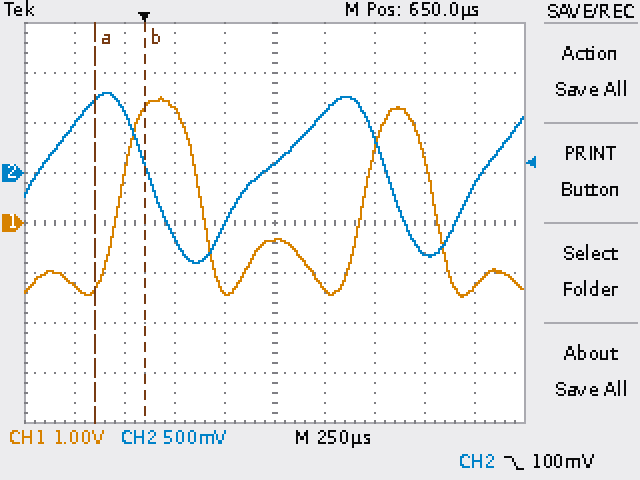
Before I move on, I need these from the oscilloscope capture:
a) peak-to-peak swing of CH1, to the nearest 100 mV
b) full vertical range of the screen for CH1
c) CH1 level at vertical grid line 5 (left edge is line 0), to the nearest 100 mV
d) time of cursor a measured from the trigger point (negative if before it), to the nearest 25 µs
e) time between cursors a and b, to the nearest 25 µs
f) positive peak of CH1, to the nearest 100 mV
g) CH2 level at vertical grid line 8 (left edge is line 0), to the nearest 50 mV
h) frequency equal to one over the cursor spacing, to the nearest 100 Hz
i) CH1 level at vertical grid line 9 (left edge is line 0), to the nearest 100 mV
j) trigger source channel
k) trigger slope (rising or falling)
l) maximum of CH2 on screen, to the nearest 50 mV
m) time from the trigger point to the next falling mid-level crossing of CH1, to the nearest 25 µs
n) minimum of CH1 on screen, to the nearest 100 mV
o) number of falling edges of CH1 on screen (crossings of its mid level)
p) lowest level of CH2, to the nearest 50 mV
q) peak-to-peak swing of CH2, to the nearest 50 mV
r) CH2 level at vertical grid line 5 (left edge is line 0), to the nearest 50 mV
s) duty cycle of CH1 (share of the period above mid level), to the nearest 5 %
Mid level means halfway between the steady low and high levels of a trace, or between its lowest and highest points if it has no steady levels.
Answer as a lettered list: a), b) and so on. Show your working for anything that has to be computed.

a) 2.5 V − (-1.5 V) = 4.0 V
b) 8 V
c) -300 mV
d) -250 µs
e) 250 µs
f) 2.5 V
g) -800 mV
h) 1 / 250 µs ≈ 4.0 kHz
i) -1.3 V
j) CH2
k) falling
l) 800 mV
m) 275 µs
n) -1.5 V
o) 2
p) -900 mV
q) 800 mV − (-900 mV) = 1.70 V
r) 100 mV
s) 30 %
